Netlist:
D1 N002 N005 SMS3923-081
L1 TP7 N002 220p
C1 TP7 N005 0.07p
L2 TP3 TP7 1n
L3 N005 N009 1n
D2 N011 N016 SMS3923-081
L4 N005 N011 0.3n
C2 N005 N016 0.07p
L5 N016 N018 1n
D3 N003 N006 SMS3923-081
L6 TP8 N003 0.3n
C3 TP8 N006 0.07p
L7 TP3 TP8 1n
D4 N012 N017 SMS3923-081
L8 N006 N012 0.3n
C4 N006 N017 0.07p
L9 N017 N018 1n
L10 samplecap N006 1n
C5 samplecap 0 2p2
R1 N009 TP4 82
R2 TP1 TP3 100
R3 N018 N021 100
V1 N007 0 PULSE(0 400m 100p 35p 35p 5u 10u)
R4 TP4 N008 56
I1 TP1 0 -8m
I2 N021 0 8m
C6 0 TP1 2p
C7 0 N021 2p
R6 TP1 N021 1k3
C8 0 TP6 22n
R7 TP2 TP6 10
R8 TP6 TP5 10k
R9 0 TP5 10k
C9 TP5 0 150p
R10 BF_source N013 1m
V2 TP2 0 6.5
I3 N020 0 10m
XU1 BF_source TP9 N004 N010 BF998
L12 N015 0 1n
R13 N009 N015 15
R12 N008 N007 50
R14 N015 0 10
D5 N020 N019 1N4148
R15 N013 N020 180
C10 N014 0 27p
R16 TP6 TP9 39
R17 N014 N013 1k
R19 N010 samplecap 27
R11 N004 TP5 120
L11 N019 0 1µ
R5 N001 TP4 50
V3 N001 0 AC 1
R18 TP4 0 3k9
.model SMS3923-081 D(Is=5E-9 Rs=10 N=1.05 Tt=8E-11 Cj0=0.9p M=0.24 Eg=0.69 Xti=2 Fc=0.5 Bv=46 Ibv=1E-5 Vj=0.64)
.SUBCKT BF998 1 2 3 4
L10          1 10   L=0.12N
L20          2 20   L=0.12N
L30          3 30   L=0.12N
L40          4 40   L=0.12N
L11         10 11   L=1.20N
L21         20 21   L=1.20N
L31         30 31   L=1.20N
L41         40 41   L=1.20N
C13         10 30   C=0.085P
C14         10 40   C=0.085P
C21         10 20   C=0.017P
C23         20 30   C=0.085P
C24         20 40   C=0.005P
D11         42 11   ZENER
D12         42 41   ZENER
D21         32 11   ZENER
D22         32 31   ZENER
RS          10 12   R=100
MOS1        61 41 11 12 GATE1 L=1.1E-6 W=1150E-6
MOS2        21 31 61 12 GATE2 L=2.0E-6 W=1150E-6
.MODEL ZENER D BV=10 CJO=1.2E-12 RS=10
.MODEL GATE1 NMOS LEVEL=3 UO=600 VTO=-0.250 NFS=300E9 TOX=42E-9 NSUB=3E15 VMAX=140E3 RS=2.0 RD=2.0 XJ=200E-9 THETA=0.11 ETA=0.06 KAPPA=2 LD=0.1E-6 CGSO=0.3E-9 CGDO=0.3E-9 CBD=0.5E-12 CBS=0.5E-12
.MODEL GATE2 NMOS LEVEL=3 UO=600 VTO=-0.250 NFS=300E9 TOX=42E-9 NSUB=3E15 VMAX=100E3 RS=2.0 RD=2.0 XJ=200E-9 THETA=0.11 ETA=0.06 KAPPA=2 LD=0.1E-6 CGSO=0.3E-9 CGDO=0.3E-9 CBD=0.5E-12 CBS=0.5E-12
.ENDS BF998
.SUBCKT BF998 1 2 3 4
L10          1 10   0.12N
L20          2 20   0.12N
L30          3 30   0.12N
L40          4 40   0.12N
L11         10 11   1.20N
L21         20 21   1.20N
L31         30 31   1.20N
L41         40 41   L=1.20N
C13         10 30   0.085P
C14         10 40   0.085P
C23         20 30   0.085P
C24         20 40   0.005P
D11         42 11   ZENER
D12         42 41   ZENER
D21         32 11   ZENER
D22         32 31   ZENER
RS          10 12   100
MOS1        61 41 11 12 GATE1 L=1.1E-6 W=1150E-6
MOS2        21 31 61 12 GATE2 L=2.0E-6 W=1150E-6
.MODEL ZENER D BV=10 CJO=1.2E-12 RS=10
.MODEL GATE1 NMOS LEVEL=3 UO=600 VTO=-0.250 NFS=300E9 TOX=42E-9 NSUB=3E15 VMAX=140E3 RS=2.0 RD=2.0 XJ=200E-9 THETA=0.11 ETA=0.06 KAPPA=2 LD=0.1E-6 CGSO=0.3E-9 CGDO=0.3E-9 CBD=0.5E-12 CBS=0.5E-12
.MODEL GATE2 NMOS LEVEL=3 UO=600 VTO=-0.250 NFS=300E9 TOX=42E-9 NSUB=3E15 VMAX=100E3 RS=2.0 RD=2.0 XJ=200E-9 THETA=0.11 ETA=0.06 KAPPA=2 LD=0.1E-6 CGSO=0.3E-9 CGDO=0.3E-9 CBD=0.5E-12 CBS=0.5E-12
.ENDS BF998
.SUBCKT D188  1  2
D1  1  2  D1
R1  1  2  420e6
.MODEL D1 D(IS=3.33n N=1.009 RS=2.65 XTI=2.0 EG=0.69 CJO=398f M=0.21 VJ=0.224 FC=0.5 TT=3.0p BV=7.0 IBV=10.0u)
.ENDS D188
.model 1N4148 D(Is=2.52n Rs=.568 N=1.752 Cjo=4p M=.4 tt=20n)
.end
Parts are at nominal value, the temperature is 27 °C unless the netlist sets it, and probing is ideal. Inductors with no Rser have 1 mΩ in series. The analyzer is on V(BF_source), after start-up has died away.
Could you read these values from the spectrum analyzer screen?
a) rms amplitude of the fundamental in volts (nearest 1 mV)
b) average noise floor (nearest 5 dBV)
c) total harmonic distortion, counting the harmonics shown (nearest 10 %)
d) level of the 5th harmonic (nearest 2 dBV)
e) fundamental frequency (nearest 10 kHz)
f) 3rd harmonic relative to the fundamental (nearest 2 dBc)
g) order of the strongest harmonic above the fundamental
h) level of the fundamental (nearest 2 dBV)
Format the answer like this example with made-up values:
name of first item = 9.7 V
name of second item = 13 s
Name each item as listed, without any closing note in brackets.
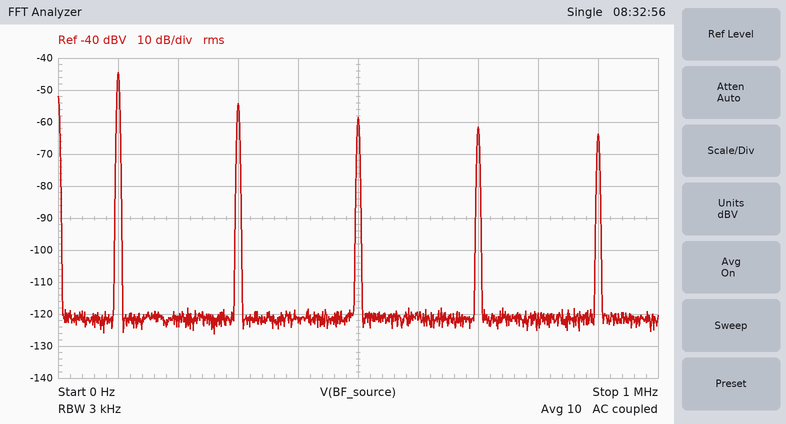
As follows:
rms amplitude of the fundamental in volts = 6 mV
average noise floor = -120 dBV
total harmonic distortion, counting the harmonics shown = 40 %
level of the 5th harmonic = -58 dBV
fundamental frequency = 100 kHz
3rd harmonic relative to the fundamental = -10 dBc
order of the strongest harmonic above the fundamental = 3
level of the fundamental = -44 dBV
